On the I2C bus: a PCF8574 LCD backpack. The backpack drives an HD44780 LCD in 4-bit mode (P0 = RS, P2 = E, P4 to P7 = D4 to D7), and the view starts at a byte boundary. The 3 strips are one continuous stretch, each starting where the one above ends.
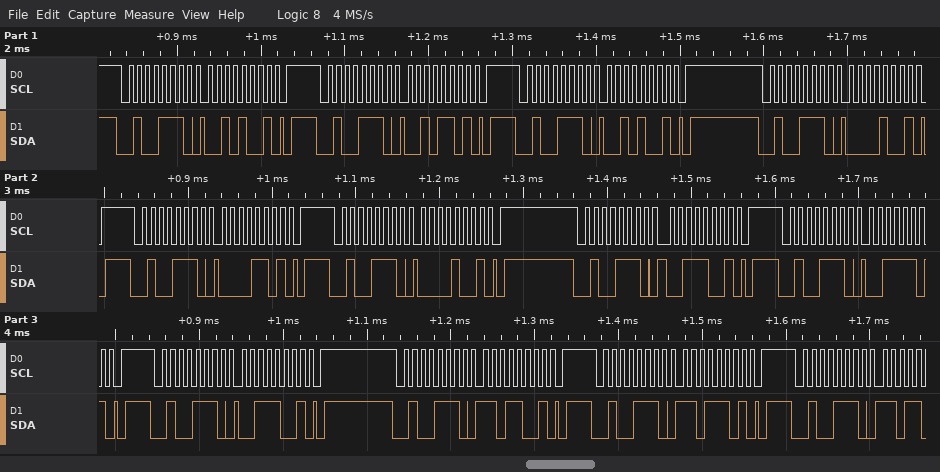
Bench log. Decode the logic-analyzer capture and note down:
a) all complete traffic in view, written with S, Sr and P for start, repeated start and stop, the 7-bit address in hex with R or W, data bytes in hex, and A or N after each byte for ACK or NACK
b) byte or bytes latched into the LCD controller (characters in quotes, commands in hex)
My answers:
S 27W A 29 A P S 27W A 2D A P S 27W A 29 A P S 27W A 09 A P S 27W A 0D A P S 27W A 09 A P S 27W A 39 A P S 27W A 3D A P S 27W A 39 A P S 27W A D9 A P S 27W A DD A P S 27W A
' '
